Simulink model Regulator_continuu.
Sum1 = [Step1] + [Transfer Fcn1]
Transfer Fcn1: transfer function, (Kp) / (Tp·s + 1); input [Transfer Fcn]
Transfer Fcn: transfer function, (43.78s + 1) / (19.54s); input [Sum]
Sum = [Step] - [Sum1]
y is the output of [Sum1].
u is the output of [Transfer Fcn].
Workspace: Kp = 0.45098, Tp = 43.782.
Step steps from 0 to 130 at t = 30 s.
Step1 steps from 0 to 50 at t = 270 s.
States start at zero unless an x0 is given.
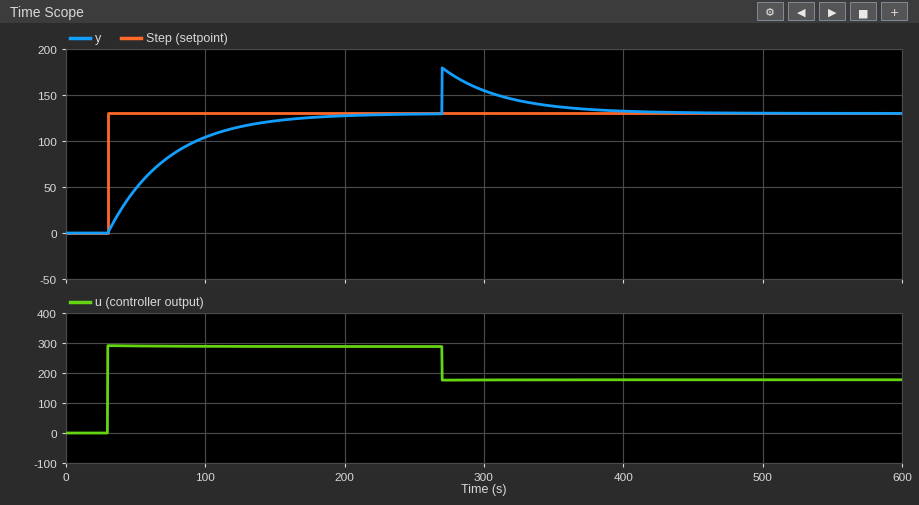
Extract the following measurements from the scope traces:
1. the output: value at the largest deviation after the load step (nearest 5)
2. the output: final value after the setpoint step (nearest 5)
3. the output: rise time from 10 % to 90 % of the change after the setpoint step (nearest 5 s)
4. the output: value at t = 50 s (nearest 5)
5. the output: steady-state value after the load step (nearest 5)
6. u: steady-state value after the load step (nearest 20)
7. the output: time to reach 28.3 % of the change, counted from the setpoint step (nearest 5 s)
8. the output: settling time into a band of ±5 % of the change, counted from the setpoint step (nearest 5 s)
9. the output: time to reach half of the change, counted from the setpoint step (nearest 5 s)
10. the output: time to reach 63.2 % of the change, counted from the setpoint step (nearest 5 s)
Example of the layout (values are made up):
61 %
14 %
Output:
180
130
95 s
50
130
180
15 s
130 s
30 s
45 s
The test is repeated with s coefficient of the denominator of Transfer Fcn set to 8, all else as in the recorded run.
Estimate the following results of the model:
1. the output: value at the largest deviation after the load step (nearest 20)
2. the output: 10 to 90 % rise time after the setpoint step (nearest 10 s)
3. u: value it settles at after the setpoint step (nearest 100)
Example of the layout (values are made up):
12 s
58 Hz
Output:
180
40 s
300
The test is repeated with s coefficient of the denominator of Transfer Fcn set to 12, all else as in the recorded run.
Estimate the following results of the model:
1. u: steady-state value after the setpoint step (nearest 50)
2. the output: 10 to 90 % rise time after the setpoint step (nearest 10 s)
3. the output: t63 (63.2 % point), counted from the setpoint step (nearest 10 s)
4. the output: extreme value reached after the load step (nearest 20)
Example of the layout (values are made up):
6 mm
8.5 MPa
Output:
300
60 s
30 s
180
